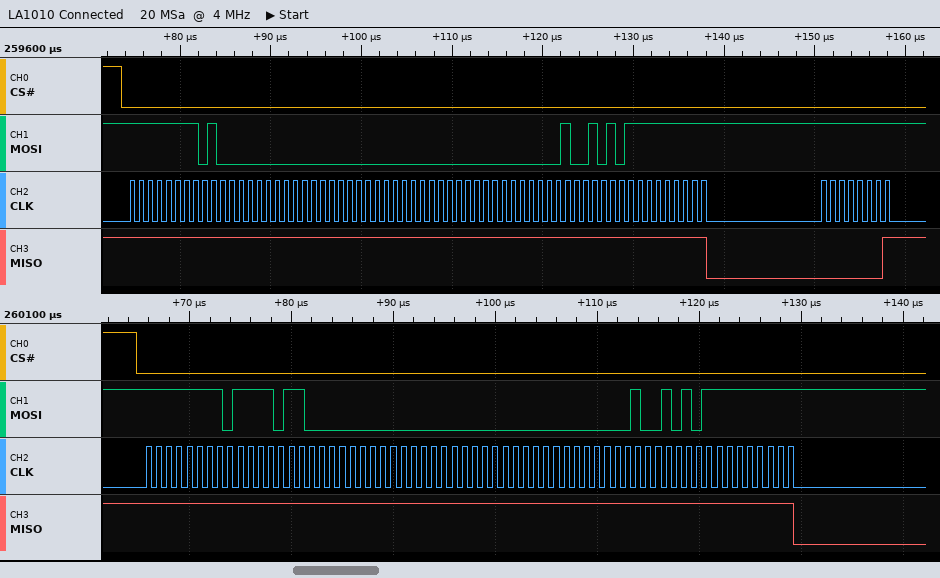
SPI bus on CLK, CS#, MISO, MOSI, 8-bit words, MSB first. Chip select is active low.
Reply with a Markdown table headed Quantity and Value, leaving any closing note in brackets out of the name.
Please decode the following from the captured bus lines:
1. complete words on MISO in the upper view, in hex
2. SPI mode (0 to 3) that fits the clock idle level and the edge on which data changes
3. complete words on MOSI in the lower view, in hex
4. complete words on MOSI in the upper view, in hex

| Quantity | Value |
|---|---|
| complete words on MISO in the upper view, in hex | FF, FF, FF, FF, FF, FF, FF, FF, 01 |
| SPI mode (0 to 3) that fits the clock idle level and the edge on which data changes | 0 |
| complete words on MOSI in the lower view, in hex | FF, 7B, 00, 00, 00, 00, 95, FF |
| complete words on MOSI in the upper view, in hex | FF, 40, 00, 00, 00, 00, 95, FF, FF |
